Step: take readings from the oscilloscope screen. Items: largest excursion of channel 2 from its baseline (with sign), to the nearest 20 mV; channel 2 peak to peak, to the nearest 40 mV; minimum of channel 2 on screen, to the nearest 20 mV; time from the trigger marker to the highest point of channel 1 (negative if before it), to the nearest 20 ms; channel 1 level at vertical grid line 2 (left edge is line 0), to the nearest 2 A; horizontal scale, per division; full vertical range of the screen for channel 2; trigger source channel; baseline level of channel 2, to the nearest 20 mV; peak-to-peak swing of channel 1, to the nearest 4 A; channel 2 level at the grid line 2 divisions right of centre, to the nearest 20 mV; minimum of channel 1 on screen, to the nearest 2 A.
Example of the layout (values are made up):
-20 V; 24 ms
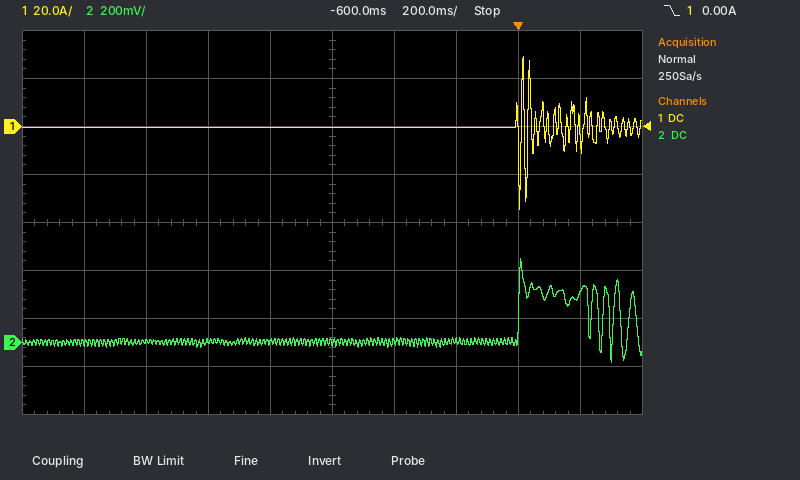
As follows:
+340 mV; 440 mV; -80 mV; +20 ms; 0 A; 200 ms; 1.6 V; channel 1; 0 mV; 64 A; 0 mV; -34 A
